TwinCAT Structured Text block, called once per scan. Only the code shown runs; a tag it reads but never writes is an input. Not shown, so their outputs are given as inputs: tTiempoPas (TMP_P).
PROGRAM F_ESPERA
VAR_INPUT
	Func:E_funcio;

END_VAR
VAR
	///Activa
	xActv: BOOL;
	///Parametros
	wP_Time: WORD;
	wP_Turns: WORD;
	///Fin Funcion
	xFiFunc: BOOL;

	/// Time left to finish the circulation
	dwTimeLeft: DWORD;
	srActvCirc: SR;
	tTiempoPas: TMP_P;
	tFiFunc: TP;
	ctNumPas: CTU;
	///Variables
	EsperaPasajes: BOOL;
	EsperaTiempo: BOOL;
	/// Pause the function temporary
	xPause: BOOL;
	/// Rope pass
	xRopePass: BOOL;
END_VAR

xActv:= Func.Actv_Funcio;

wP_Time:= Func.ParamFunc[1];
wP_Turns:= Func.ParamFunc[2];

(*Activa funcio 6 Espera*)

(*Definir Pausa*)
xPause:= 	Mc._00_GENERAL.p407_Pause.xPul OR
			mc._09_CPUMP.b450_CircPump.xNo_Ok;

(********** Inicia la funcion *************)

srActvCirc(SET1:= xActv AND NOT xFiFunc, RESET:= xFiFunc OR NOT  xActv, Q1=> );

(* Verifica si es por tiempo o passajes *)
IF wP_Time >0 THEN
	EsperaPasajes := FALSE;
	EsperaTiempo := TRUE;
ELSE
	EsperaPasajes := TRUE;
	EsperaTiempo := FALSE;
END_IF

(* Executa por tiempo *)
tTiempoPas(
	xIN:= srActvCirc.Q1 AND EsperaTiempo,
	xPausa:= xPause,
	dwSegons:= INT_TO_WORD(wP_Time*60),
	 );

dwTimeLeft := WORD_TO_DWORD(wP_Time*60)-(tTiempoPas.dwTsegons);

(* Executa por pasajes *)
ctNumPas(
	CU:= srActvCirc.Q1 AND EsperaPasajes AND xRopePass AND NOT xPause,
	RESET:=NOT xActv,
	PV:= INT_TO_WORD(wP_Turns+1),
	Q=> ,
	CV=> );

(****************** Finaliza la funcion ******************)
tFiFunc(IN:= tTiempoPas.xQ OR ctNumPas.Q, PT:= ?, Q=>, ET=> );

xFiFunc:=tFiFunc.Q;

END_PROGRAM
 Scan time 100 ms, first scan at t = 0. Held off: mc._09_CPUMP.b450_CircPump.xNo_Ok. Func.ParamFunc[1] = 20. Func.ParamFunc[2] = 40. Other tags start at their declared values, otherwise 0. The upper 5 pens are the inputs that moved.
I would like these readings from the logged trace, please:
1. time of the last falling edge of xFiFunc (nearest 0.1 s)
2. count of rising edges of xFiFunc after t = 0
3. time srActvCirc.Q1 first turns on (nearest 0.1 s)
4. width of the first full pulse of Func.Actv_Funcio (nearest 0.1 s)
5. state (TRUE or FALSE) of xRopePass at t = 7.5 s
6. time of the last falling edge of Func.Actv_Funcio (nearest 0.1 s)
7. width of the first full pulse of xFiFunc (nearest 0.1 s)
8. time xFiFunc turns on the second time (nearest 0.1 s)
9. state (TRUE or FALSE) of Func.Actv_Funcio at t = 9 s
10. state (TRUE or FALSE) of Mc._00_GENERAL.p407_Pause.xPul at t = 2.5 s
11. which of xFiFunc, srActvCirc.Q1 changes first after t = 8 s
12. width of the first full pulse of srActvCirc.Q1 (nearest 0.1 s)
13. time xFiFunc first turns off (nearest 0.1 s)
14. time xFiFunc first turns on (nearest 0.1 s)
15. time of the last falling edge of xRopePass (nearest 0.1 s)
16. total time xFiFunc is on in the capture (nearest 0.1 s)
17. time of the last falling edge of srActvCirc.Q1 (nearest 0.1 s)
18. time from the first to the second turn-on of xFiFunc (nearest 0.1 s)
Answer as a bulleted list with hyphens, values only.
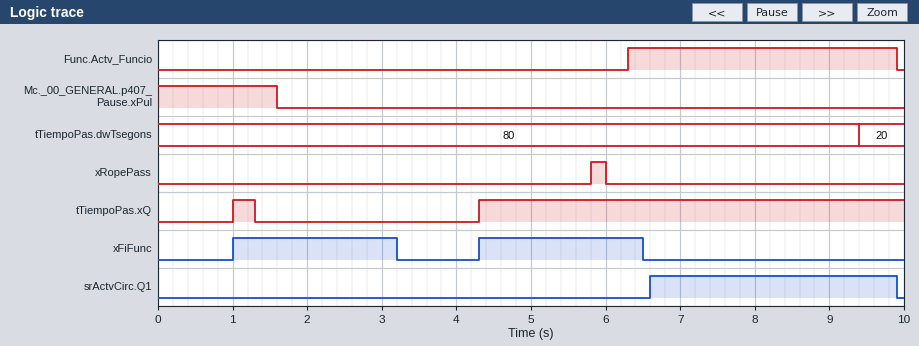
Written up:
- 6.5 s
- 2
- 6.6 s
- 3.6 s
- FALSE
- 9.9 s
- 2.2 s
- 4.3 s
- TRUE
- FALSE
- srActvCirc.Q1
- 3.3 s
- 3.2 s
- 1.0 s
- 6.0 s
- 4.4 s
- 9.9 s
- 3.3 s
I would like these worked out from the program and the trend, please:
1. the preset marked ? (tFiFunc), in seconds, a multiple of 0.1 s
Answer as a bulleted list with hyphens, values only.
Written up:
- 2.2 s
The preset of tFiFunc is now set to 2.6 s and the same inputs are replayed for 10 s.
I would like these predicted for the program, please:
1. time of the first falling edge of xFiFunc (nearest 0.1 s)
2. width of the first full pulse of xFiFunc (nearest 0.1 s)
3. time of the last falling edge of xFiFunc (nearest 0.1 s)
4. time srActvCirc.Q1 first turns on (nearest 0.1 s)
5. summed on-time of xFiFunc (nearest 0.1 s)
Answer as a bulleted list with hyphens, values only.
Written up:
- 3.6 s
- 2.6 s
- 6.9 s
- 7.0 s
- 5.2 s
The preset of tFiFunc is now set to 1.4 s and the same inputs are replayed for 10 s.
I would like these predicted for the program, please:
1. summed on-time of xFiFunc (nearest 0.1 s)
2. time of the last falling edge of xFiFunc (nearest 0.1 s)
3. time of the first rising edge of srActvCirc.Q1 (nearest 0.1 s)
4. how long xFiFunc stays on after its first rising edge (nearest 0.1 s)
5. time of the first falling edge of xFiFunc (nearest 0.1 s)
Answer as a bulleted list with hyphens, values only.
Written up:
- 2.8 s
- 5.7 s
- 6.3 s
- 1.4 s
- 2.4 s
